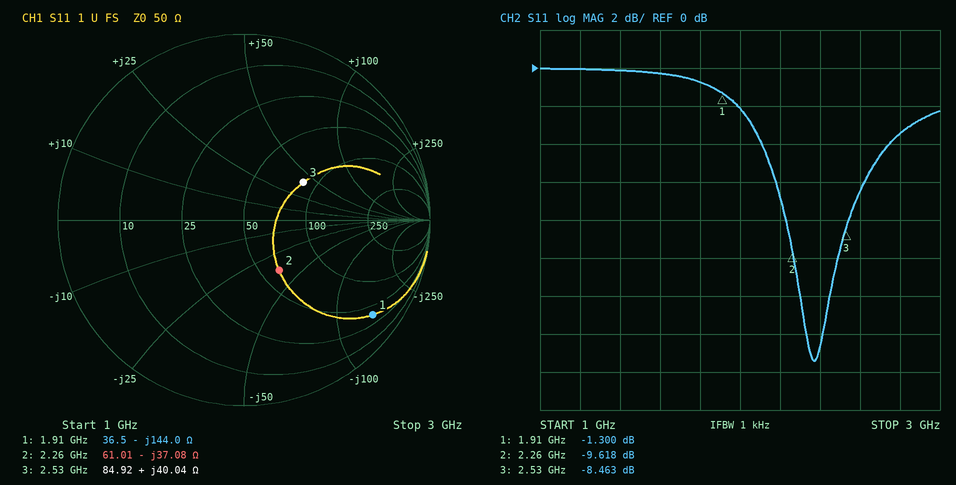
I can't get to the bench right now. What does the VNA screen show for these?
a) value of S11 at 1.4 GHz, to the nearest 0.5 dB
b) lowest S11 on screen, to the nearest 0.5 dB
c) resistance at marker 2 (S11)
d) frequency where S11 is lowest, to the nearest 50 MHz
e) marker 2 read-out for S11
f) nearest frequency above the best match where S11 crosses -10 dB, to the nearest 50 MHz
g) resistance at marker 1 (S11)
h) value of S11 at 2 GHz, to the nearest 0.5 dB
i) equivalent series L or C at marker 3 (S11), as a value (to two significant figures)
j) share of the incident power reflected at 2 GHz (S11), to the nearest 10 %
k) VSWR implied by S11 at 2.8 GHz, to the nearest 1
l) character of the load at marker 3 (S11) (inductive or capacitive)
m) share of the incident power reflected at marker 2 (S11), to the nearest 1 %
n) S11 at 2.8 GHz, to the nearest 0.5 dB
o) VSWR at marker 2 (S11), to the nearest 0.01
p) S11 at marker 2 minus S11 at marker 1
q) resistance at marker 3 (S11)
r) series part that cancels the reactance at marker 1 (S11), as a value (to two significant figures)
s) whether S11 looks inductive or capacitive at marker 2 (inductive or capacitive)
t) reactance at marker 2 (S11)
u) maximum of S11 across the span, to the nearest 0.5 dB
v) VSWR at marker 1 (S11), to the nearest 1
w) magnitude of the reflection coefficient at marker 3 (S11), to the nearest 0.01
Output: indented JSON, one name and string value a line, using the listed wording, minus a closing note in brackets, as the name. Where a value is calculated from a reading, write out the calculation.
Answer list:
{
  "value of S11 at 1.4 GHz, to the nearest 0.5 dB": "0.0 dB",
  "lowest S11 on screen, to the nearest 0.5 dB": "-15.5 dB",
  "resistance at marker 2": "61.01 Ω",
  "frequency where S11 is lowest, to the nearest 50 MHz": "2.35 GHz",
  "marker 2 read-out for S11": "-9.618 dB",
  "nearest frequency above the best match where S11 crosses -10 dB, to the nearest 50 MHz": "2.50 GHz",
  "resistance at marker 1": "36.5 Ω",
  "value of S11 at 2 GHz, to the nearest 0.5 dB": "-2.0 dB",
  "equivalent series L or C at marker 3 (S11), as a value": "L = 40.04 Ω/(2π × 2.53 GHz) ≈ 2.5 nH",
  "share of the incident power reflected at 2 GHz (S11), to the nearest 10 %": "10^(-2/10) ≈ 63.1 %, so 60 % to the nearest 10 %",
  "VSWR implied by S11 at 2.8 GHz, to the nearest 1": "|Γ| = 10^(-3.5/20) = 0.6683; VSWR = (1 + 0.6683)/(1 − 0.6683) ≈ 5",
  "character of the load at marker 3 (S11)": "inductive",
  "share of the incident power reflected at marker 2 (S11), to the nearest 1 %": "10^(-9.618/10) ≈ 11 %",
  "S11 at 2.8 GHz, to the nearest 0.5 dB": "-3.5 dB",
  "VSWR at marker 2 (S11), to the nearest 0.01": "1.99",
  "S11 at marker 2 minus S11 at marker 1": "-9.618 − (-1.3) = -8.318 dB",
  "resistance at marker 3": "84.92 Ω",
  "series part that cancels the reactance at marker 1 (S11), as a value": "L = 144 Ω/(2π × 1.91 GHz) ≈ 12 nH",
  "whether S11 looks inductive or capacitive at marker 2": "capacitive",
  "reactance at marker 2": "-37.08 Ω",
  "maximum of S11 across the span, to the nearest 0.5 dB": "0.0 dB",
  "VSWR at marker 1 (S11), to the nearest 1": "13",
  "magnitude of the reflection coefficient at marker 3 (S11), to the nearest 0.01": "0.38"
}
